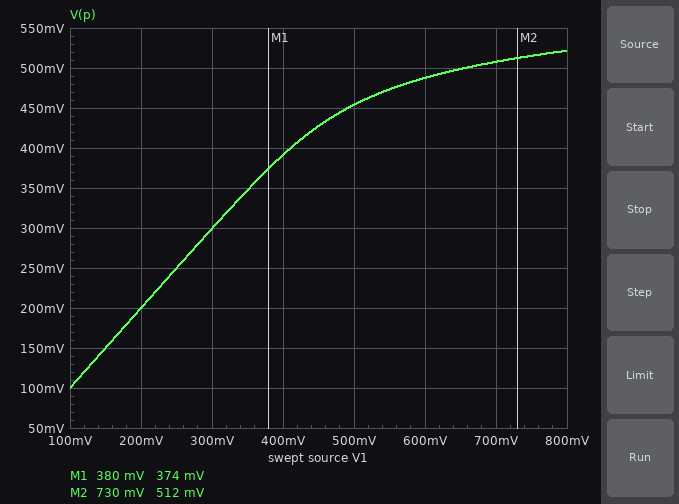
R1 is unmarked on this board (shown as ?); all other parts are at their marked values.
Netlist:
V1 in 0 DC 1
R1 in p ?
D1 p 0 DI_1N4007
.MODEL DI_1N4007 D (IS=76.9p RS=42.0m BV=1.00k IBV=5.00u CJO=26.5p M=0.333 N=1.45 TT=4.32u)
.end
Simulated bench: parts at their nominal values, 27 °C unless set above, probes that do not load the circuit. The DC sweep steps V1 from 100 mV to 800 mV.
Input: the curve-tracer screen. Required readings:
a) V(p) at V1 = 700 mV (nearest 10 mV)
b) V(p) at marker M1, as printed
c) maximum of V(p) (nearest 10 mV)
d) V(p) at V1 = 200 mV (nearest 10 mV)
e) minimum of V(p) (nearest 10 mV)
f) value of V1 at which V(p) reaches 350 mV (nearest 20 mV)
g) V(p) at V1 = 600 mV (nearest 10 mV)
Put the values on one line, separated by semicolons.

510 mV; 374 mV; 520 mV; 200 mV; 100 mV; 360 mV; 490 mV
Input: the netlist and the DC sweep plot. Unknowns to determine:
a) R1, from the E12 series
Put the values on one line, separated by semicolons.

3.3 kΩ
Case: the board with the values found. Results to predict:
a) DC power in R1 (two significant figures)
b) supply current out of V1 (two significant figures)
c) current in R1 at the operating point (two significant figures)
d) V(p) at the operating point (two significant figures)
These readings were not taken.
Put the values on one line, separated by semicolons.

64 µW; 140 µA; 140 µA; 540 mV
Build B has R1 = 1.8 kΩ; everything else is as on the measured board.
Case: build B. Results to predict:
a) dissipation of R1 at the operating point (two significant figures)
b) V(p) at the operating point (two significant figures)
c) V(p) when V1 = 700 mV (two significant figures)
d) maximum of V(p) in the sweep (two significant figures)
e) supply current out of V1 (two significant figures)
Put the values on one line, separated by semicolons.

110 µW; 560 mV; 530 mV; 540 mV; 240 µA
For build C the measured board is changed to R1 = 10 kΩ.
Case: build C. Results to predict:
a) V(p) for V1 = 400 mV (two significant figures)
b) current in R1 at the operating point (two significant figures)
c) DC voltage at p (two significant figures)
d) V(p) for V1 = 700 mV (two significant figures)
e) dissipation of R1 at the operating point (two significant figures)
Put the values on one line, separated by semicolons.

380 mV; 50 µA; 500 mV; 470 mV; 25 µW
